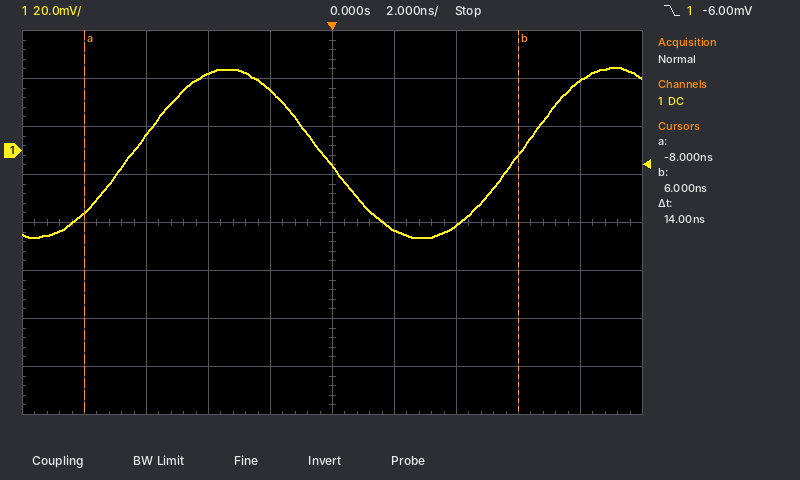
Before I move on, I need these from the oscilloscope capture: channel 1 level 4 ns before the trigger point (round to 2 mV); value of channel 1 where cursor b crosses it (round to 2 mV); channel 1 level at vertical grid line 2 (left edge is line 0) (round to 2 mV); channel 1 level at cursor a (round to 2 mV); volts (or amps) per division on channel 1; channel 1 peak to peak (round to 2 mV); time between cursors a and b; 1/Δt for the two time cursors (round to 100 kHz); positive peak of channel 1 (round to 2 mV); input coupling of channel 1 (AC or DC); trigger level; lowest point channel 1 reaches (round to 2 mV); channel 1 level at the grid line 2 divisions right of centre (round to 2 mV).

32 mV
-2 mV
6 mV
-26 mV
20 mV
70 mV
14 ns
71.4 MHz
34 mV
DC
-6.00 mV
-36 mV
-32 mV
